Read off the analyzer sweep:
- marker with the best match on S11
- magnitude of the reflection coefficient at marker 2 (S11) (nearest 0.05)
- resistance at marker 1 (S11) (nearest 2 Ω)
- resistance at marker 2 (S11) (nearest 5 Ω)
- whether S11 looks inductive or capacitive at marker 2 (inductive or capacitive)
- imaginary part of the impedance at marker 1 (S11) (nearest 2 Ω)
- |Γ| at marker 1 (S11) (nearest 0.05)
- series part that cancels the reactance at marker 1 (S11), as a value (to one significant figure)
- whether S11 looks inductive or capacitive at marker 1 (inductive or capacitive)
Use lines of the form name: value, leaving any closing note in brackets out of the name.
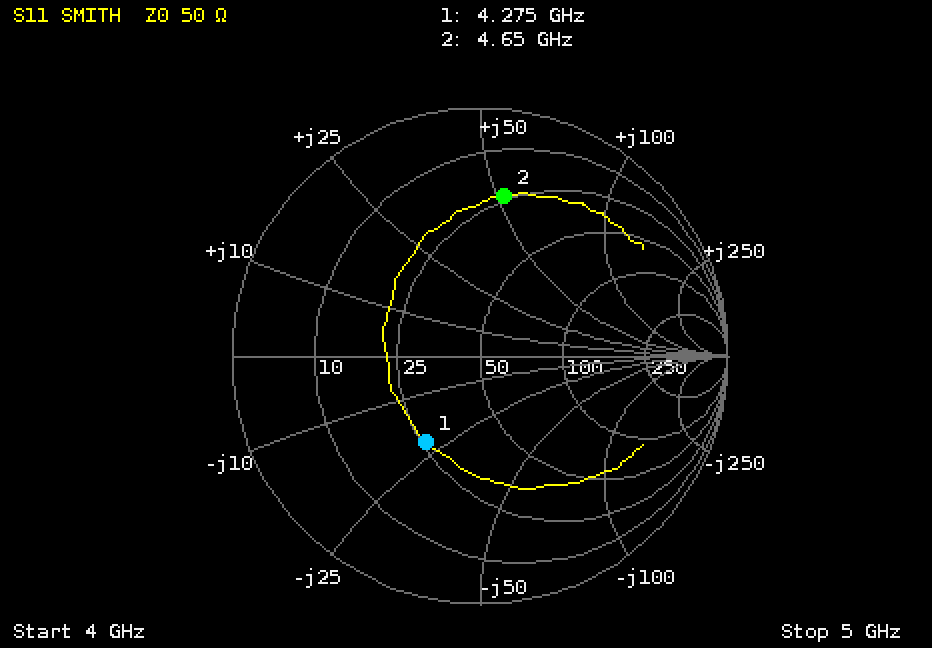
marker with the best match on S11: marker 1
magnitude of the reflection coefficient at marker 2 (S11): 0.65
resistance at marker 1 (S11): 26 Ω
resistance at marker 2 (S11): 25 Ω
whether S11 looks inductive or capacitive at marker 2: inductive
imaginary part of the impedance at marker 1 (S11): -22 Ω
|Γ| at marker 1 (S11): 0.40
series part that cancels the reactance at marker 1 (S11), as a value: 800 pH
whether S11 looks inductive or capacitive at marker 1: capacitive
